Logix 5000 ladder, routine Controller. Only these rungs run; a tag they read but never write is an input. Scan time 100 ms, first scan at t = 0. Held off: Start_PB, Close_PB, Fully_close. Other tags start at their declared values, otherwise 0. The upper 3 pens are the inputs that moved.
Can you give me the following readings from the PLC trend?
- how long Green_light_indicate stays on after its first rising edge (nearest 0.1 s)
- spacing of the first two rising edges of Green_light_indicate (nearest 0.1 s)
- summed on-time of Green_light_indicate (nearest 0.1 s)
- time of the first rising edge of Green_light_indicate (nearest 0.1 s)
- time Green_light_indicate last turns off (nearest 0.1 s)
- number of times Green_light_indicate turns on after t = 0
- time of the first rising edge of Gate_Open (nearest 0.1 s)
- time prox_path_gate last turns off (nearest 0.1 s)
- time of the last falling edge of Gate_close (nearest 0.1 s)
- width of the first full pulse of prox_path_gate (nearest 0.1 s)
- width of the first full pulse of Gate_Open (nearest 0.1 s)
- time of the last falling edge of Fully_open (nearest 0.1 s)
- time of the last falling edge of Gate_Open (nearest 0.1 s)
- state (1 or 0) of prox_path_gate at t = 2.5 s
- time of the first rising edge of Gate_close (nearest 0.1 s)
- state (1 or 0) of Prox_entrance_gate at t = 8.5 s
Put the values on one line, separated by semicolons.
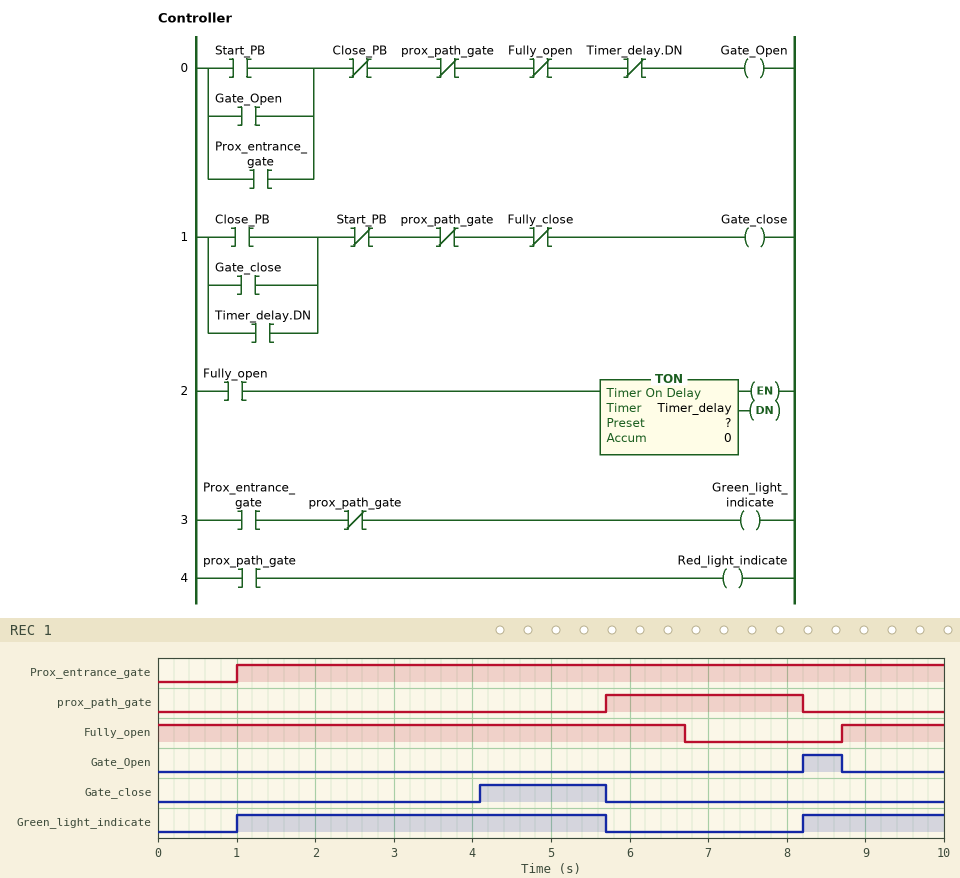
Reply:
4.7 s; 7.2 s; 6.5 s; 1.0 s; 5.7 s; 2; 8.2 s; 8.2 s; 5.7 s; 2.5 s; 0.5 s; 6.7 s; 8.7 s; 0; 4.1 s; 1
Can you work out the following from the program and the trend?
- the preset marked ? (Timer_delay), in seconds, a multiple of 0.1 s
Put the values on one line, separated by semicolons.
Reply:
4.0 s
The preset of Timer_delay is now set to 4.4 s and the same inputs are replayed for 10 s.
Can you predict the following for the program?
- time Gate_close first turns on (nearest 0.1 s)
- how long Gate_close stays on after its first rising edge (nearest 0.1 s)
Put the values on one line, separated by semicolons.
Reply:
4.5 s; 1.2 s
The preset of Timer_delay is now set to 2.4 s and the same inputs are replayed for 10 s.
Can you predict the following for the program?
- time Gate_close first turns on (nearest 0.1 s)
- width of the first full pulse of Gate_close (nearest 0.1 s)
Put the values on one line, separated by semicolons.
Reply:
2.5 s; 3.2 s
